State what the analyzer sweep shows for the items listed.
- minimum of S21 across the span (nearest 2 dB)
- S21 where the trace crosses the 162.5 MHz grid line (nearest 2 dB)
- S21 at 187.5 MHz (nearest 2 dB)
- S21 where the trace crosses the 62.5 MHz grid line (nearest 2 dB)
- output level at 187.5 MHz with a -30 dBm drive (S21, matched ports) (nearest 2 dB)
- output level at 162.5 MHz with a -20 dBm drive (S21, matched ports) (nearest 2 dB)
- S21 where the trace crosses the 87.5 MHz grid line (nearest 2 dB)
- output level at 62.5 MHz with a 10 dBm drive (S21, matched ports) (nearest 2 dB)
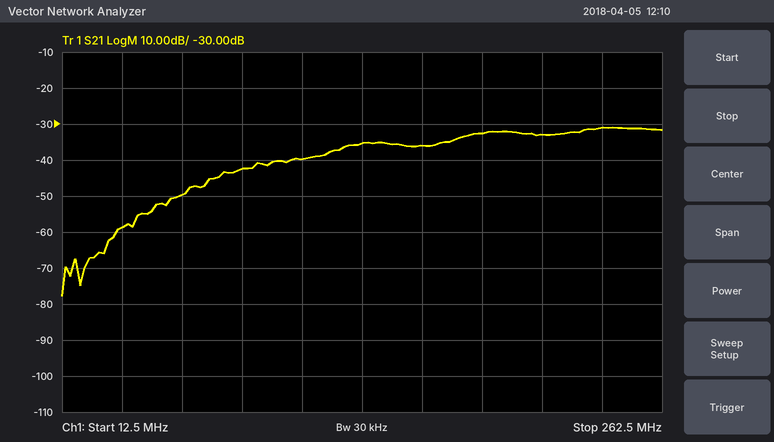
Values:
-78 dB
-36 dB
-32 dB
-50 dB
-62 dBm
-56 dBm
-42 dB
-40 dBm
